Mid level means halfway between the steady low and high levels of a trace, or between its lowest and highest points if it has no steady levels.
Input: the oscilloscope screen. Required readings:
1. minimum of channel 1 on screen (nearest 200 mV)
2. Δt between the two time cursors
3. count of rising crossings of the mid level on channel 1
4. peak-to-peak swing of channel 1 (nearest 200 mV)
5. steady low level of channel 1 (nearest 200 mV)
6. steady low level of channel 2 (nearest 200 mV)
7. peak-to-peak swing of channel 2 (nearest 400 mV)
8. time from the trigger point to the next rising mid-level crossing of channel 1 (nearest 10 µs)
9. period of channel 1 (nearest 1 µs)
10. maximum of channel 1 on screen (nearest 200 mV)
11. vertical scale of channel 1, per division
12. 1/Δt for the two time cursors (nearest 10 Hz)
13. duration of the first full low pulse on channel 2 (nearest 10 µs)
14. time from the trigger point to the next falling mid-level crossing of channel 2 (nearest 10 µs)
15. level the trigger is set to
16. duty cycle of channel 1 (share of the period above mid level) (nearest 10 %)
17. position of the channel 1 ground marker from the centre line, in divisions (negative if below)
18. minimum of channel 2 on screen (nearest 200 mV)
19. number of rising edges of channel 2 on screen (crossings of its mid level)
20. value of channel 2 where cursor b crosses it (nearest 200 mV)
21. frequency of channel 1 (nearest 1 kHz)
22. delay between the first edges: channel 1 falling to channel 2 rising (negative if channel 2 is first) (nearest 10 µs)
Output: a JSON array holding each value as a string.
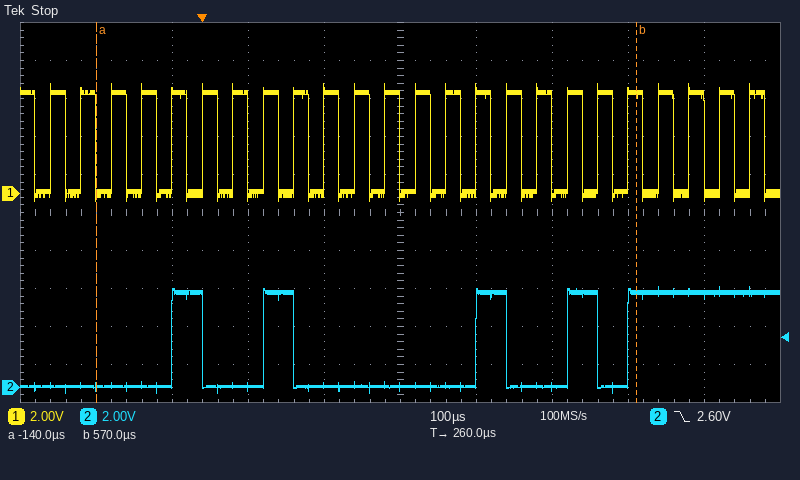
["-400 mV", "710 µs", "24", "6.2 V", "0.0 V", "0.0 V", "5.6 V", "40 µs", "40 µs", "5.8 V", "2 V", "1.41 kHz", "80 µs", "120 µs", "2.60 V", "50 %", "+0.5 div", "-400 mV", "5", "5.0 V", "25 kHz", "+180 µs"]
